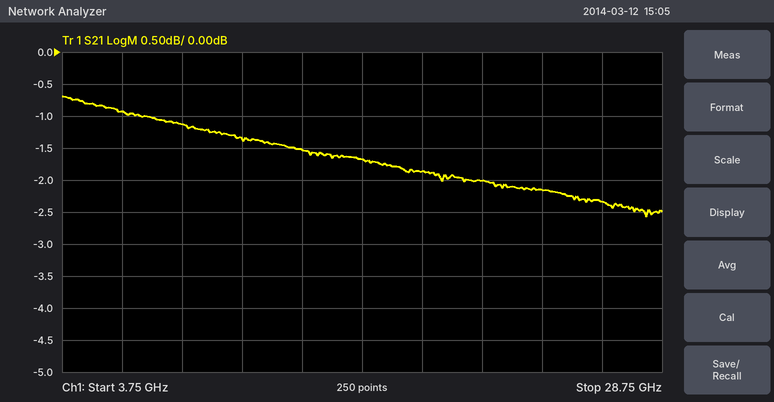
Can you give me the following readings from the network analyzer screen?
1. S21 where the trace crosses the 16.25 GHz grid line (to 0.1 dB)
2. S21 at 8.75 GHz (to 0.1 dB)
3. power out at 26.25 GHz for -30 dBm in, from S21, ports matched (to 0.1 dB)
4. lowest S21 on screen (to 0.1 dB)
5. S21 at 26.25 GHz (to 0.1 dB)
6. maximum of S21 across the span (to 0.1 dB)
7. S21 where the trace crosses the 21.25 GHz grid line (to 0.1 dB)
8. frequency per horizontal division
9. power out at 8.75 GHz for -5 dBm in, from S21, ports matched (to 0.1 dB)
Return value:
-1.7 dB
-1.1 dB
-32.3 dBm
-2.6 dB
-2.3 dB
-0.7 dB
-2.0 dB
2.5 GHz
-6.1 dBm
